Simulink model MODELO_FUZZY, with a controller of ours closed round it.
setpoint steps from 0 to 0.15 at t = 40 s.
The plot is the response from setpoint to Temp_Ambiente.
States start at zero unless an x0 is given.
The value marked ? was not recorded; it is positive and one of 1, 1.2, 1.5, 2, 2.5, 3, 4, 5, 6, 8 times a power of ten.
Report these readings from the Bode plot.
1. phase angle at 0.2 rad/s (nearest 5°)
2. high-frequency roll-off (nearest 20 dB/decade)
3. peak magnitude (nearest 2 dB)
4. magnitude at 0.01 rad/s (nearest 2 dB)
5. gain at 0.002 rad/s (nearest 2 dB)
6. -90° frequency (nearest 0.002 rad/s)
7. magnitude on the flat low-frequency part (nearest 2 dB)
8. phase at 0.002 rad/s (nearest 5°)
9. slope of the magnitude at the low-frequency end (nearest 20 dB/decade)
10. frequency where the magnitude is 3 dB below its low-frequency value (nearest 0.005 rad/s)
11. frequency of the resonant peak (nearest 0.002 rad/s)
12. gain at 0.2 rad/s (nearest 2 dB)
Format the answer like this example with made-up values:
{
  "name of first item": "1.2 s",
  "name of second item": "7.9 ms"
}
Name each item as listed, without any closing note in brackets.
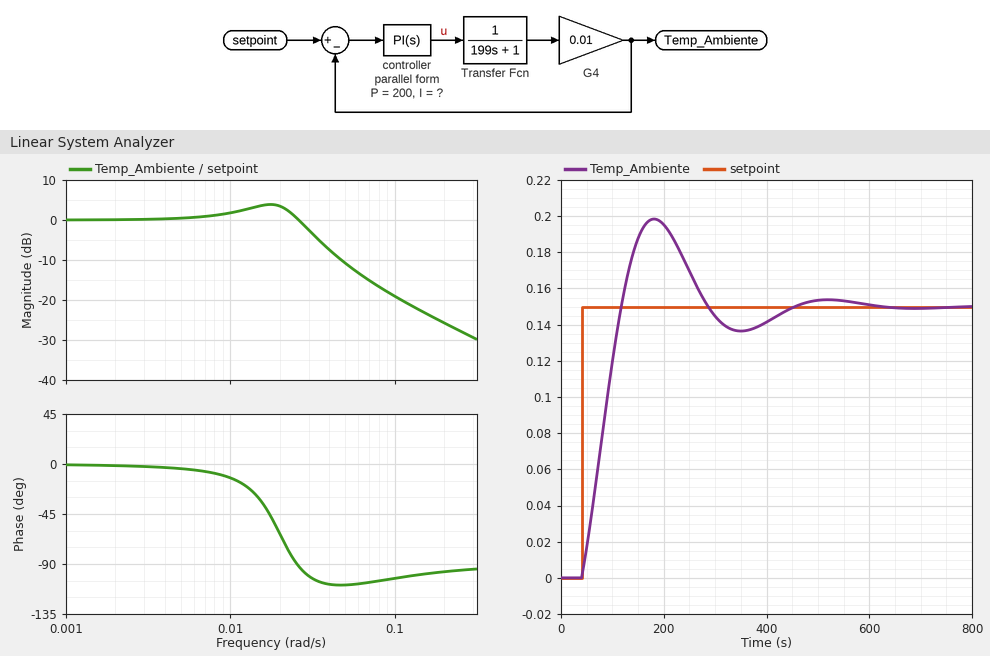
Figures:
{
  "phase angle at 0.2 rad/s": "-95°",
  "high-frequency roll-off": "-20 dB/decade",
  "peak magnitude": "4 dB",
  "magnitude at 0.01 rad/s": "2 dB",
  "gain at 0.002 rad/s": "0 dB",
  "-90° frequency": "0.026 rad/s",
  "magnitude on the flat low-frequency part": "0 dB",
  "phase at 0.002 rad/s": "0°",
  "slope of the magnitude at the low-frequency end": "0 dB/decade",
  "frequency where the magnitude is 3 dB below its low-frequency value": "0.030 rad/s",
  "frequency of the resonant peak": "0.018 rad/s",
  "gain at 0.2 rad/s": "-26 dB"
}
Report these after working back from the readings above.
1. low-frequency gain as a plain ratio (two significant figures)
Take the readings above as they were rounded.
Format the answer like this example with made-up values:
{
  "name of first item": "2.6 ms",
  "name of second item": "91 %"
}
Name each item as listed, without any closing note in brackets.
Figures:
{
  "low-frequency gain as a plain ratio": "1.0"
}
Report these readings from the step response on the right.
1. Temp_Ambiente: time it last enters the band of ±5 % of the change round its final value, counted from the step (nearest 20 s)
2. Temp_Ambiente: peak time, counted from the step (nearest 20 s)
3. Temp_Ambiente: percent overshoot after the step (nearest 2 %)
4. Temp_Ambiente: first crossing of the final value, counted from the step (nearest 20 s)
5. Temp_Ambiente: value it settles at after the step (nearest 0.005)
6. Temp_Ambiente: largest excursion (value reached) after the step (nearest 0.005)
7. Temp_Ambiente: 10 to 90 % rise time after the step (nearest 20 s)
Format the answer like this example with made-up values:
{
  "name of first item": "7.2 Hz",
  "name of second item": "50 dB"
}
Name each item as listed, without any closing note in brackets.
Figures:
{
  "Temp_Ambiente: time it last enters the band of ±5 % of the change round its final value, counted from the step": "360 s",
  "Temp_Ambiente: peak time, counted from the step": "140 s",
  "Temp_Ambiente: percent overshoot after the step": "32 %",
  "Temp_Ambiente: first crossing of the final value, counted from the step": "80 s",
  "Temp_Ambiente: value it settles at after the step": "0.150",
  "Temp_Ambiente: largest excursion (value reached) after the step": "0.200",
  "Temp_Ambiente: 10 to 90 % rise time after the step": "60 s"
}
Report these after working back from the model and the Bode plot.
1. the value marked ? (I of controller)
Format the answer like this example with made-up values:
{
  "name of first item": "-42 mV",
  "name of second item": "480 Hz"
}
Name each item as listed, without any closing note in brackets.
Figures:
{
  "the value marked ?": "8"
}
